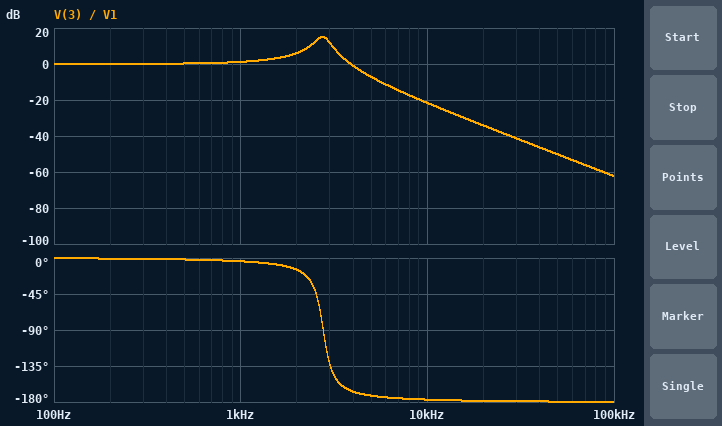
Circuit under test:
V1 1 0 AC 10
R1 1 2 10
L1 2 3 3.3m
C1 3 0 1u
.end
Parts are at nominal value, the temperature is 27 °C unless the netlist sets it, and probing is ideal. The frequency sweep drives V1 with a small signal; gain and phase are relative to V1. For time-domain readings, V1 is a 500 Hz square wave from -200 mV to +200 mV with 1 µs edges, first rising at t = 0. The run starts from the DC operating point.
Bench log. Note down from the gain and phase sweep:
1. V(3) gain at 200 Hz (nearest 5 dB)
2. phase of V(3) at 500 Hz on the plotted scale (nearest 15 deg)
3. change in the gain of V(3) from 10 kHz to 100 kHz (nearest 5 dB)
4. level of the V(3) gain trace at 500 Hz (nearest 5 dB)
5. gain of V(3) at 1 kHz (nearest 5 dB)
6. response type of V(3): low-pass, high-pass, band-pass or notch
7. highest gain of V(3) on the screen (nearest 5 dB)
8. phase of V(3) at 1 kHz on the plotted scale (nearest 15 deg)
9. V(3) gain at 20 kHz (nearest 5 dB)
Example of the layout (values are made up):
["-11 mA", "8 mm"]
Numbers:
["0 dB", "0 deg", "-40 dB", "0 dB", "0 dB", "low-pass", "15 dB", "0 deg", "-35 dB"]
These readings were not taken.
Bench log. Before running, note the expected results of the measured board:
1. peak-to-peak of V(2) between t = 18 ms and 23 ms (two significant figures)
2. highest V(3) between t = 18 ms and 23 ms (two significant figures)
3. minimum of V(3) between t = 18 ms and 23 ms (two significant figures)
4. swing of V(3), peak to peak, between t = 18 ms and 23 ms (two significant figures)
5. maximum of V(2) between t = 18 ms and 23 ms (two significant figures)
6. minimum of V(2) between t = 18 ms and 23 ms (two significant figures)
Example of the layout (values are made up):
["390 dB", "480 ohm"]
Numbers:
["490 mV", "500 mV", "-500 mV", "1.0 V", "250 mV", "-250 mV"]
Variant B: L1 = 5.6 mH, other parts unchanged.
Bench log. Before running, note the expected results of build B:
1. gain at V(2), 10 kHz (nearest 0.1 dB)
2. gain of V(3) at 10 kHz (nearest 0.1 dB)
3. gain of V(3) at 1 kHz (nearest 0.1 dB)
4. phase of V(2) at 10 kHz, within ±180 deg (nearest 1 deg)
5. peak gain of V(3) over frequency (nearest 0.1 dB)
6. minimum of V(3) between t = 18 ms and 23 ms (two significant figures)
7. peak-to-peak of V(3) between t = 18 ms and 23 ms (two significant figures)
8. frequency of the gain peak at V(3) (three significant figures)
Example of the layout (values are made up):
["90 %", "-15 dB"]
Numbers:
["0 dB", "-26.5 dB", "2.1 dB", "2 deg", "17.5 dB", "-440 mV", "880 mV", "2.12 kHz"]
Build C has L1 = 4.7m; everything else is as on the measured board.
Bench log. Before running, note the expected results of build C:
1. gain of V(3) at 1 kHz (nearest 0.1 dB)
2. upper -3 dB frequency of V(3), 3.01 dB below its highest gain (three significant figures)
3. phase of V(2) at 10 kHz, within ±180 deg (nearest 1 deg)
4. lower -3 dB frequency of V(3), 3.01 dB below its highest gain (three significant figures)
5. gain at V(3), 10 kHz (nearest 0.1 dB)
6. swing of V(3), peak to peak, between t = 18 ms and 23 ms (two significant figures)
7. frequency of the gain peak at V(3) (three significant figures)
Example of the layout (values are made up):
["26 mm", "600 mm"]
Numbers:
["1.8 dB", "2.47 kHz", "2 deg", "2.13 kHz", "-24.9 dB", "1.1 V", "2.31 kHz"]
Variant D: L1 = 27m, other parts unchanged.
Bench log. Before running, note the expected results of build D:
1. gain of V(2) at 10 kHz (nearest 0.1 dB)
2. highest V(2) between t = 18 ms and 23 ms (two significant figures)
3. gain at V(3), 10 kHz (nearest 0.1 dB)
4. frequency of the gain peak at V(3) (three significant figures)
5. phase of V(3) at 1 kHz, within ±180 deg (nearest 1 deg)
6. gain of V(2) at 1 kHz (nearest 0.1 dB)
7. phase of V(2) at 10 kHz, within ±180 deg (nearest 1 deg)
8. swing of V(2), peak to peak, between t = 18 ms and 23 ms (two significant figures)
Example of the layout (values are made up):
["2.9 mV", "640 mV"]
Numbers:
["0 dB", "210 mV", "-40.5 dB", "968 Hz", "-136 deg", "-2.8 dB", "0 deg", "420 mV"]
